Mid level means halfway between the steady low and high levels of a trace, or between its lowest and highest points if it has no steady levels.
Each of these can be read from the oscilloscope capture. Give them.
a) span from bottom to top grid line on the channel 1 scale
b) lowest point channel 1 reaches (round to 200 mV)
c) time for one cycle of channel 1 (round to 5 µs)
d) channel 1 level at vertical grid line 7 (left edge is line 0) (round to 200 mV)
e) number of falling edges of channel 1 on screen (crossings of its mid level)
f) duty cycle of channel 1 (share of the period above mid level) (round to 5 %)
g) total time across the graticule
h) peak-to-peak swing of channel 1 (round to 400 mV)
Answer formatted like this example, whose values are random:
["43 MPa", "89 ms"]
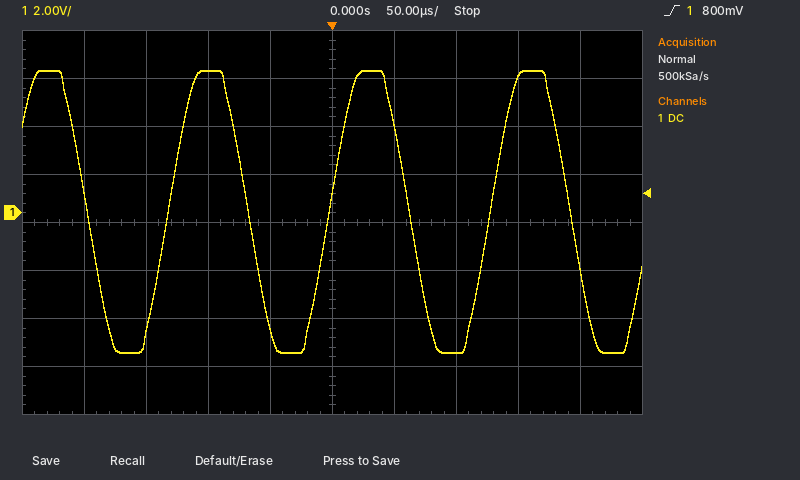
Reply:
["16 V", "-5.8 V", "130 µs", "-5.8 V", "4", "50 %", "500 µs", "11.6 V"]
